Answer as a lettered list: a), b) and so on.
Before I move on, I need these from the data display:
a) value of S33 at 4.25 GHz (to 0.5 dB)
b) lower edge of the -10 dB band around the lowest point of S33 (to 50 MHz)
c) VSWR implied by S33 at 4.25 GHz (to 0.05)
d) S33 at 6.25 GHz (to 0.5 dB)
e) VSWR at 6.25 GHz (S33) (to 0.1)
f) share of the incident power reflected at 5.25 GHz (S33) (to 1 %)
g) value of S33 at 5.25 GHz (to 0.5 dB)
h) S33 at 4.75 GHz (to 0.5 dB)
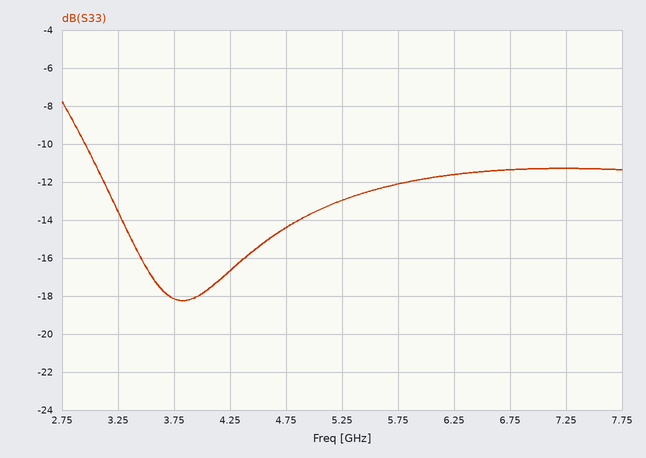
a) -16.5 dB
b) 2.95 GHz
c) 1.35
d) -11.5 dB
e) 1.7
f) 5 %
g) -13.0 dB
h) -14.5 dB
